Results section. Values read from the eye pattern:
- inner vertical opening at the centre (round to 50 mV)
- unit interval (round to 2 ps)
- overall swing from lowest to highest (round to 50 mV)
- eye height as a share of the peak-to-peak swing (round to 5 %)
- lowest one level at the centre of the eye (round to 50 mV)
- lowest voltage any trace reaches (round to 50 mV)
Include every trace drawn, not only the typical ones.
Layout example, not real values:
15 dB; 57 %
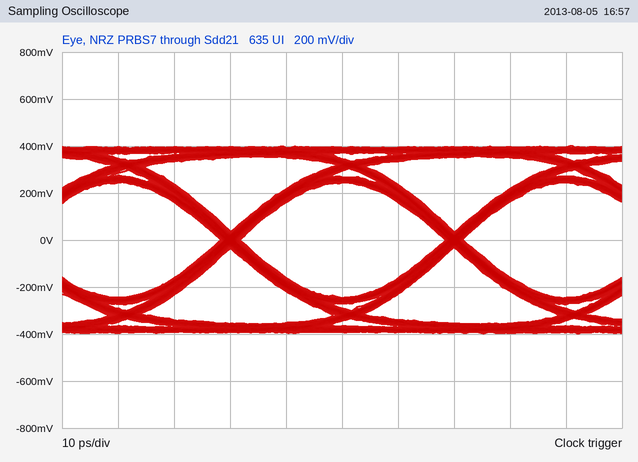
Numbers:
500 mV; 40 ps; 800 mV; 60 %; 250 mV; -400 mV
